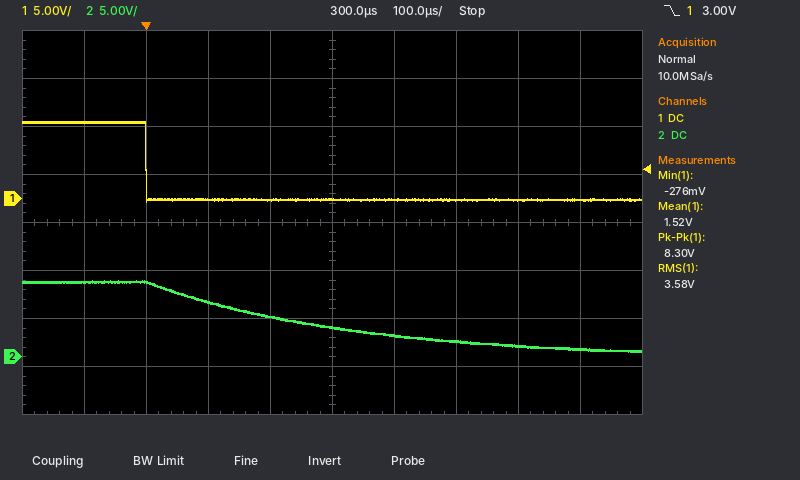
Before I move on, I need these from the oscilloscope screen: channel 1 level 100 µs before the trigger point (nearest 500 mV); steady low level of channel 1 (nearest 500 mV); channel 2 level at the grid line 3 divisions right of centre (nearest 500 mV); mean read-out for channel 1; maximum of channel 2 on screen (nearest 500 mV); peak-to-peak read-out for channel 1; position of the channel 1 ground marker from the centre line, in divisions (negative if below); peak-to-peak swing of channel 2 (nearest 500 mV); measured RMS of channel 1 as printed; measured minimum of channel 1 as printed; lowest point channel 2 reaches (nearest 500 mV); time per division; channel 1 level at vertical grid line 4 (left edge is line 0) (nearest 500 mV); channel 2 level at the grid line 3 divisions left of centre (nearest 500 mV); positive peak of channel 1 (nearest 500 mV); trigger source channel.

8.0 V
0.0 V
1.0 V
1.52 V
8.0 V
8.30 V
+0.5 div
7.5 V
3.58 V
-276 mV
500 mV
100 µs
0.0 V
8.0 V
8.0 V
channel 1
